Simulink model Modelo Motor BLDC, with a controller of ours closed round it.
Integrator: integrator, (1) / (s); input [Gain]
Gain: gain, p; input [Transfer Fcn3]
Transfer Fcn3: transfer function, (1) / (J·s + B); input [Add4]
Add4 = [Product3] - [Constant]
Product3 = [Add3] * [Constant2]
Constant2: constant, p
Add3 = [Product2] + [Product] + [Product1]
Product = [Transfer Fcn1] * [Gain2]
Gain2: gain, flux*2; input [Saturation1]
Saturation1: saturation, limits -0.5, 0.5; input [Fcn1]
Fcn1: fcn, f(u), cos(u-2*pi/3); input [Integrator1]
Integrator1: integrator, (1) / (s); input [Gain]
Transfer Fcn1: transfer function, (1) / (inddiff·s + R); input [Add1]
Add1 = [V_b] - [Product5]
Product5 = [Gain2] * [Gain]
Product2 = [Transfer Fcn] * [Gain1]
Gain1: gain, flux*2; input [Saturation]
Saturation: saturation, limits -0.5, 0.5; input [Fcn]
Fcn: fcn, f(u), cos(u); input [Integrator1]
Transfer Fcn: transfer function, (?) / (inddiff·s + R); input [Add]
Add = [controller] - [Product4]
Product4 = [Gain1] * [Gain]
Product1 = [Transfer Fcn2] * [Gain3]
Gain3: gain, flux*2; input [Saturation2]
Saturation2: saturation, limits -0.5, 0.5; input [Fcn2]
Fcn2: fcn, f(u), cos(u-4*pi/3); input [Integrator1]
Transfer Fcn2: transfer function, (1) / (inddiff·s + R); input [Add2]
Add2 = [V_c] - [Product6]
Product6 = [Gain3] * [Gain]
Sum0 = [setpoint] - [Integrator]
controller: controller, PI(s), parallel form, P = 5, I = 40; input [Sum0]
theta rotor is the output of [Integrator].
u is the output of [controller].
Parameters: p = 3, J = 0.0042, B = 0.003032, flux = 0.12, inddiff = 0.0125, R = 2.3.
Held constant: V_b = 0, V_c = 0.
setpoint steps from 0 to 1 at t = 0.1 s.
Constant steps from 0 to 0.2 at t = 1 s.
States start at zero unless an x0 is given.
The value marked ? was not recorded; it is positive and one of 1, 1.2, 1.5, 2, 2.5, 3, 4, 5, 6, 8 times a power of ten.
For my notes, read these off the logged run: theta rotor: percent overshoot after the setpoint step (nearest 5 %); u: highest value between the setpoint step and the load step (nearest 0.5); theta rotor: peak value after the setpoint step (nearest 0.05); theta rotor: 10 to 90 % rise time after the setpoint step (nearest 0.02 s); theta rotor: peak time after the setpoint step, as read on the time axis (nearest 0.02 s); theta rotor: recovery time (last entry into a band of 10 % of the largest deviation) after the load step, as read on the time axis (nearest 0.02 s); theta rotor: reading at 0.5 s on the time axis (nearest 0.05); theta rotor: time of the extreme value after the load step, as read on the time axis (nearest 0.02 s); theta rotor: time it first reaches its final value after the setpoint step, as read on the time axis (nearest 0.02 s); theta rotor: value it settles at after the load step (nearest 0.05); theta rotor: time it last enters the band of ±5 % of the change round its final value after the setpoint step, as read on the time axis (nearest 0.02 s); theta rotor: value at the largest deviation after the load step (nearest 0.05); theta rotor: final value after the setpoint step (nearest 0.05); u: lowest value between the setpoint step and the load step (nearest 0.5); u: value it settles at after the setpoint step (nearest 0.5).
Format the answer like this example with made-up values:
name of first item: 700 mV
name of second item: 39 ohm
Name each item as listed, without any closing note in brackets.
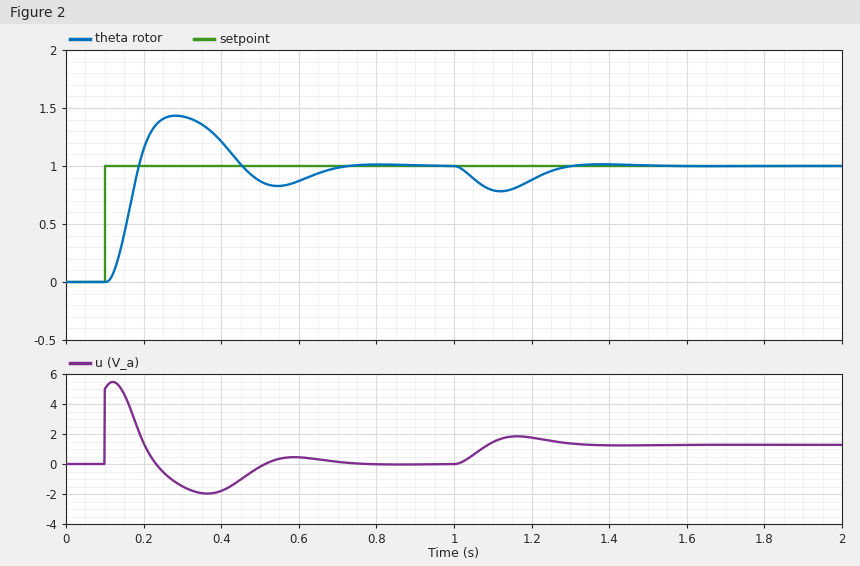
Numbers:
theta rotor: percent overshoot after the setpoint step: 45 %
u: highest value between the setpoint step and the load step: 5.5
theta rotor: peak value after the setpoint step: 1.45
theta rotor: 10 to 90 % rise time after the setpoint step: 0.06 s
theta rotor: peak time after the setpoint step, as read on the time axis: 0.28 s
theta rotor: recovery time (last entry into a band of 10 % of the largest deviation) after the load step, as read on the time axis: 1.28 s
theta rotor: reading at 0.5 s on the time axis: 0.85
theta rotor: time of the extreme value after the load step, as read on the time axis: 1.12 s
theta rotor: time it first reaches its final value after the setpoint step, as read on the time axis: 0.18 s
theta rotor: value it settles at after the load step: 1.00
theta rotor: time it last enters the band of ±5 % of the change round its final value after the setpoint step, as read on the time axis: 0.66 s
theta rotor: value at the largest deviation after the load step: 0.80
theta rotor: final value after the setpoint step: 1.00
u: lowest value between the setpoint step and the load step: -2.0
u: value it settles at after the setpoint step: 0.0
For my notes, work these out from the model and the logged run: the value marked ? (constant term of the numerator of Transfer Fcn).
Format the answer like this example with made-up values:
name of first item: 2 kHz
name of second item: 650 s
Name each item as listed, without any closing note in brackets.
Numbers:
the value marked ?: 1
